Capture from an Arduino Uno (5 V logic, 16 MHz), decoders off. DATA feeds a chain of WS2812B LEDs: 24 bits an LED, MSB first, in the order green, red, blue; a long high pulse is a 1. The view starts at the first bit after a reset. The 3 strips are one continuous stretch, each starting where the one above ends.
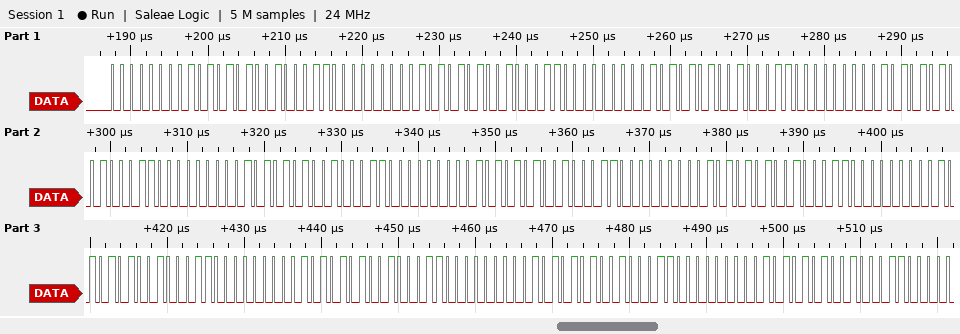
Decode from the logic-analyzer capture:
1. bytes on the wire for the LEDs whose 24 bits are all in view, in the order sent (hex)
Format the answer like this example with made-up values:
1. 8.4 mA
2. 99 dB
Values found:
1. 00 AA 46 00 AA 46 00 AA 46 00 AA 46 00 AA 46 00 AA 46 00 AA 46 00 AA 46 00 AA 46 00 AA 46 00 AA 46
